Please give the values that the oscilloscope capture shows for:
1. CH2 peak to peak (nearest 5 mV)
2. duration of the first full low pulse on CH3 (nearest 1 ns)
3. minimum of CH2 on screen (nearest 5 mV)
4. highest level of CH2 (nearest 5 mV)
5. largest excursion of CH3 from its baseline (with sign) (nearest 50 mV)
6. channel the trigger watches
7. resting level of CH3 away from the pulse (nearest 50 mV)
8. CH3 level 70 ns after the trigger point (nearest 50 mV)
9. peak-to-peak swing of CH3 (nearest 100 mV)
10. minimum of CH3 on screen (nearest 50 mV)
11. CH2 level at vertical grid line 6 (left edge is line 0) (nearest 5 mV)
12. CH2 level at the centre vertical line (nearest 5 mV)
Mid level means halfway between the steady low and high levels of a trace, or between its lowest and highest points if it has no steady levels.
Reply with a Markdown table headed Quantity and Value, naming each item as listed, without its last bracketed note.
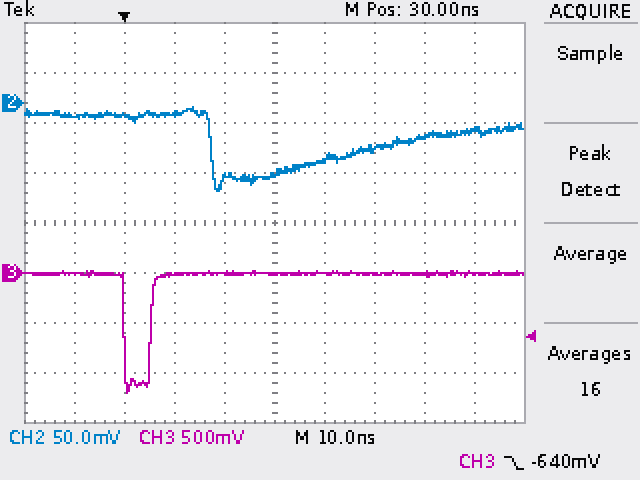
| Quantity | Value |
|---|---|
| CH2 peak to peak | 85 mV |
| duration of the first full low pulse on CH3 | 5 ns |
| minimum of CH2 on screen | -90 mV |
| highest level of CH2 | -5 mV |
| largest excursion of CH3 from its baseline (with sign) | -1.20 V |
| channel the trigger watches | CH3 |
| resting level of CH3 away from the pulse | 0 mV |
| CH3 level 70 ns after the trigger point | 0 mV |
| peak-to-peak swing of CH3 | 1.20 V |
| minimum of CH3 on screen | -1.20 V |
| CH2 level at vertical grid line 6 (left edge is line 0) | -55 mV |
| CH2 level at the centre vertical line | -70 mV |
